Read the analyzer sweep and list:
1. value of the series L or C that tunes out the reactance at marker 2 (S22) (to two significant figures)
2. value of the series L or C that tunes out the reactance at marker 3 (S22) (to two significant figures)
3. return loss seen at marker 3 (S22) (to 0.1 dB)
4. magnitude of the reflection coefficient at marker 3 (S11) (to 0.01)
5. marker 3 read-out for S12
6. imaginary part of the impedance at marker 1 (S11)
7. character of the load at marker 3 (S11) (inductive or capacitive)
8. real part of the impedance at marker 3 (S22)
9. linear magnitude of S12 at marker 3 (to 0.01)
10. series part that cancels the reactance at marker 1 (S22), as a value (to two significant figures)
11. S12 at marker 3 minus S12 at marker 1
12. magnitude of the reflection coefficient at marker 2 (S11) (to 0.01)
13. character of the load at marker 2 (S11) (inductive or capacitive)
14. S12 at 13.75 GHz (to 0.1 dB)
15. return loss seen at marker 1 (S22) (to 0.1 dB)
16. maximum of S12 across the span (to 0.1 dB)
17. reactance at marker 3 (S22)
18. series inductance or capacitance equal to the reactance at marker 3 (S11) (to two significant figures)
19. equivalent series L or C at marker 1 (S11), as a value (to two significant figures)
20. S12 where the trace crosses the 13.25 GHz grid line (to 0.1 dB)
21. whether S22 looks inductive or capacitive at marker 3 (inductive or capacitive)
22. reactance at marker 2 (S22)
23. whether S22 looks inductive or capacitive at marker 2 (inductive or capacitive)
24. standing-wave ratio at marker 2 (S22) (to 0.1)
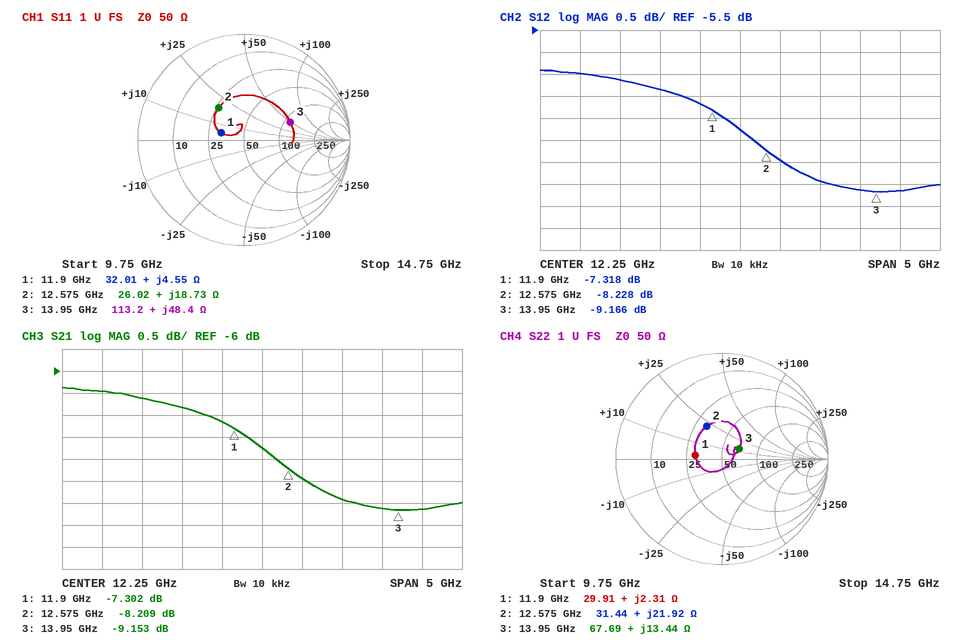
580 fF
850 fF
14.5 dB
0.47
-9.166 dB
+4.55 Ω
inductive
67.69 Ω
0.35
5.8 pF
-1.848 dB
0.39
inductive
-9.1 dB
11.9 dB
-6.4 dB
+13.44 Ω
550 pH
61 pH
-8.9 dB
inductive
+21.92 Ω
inductive
2.0
